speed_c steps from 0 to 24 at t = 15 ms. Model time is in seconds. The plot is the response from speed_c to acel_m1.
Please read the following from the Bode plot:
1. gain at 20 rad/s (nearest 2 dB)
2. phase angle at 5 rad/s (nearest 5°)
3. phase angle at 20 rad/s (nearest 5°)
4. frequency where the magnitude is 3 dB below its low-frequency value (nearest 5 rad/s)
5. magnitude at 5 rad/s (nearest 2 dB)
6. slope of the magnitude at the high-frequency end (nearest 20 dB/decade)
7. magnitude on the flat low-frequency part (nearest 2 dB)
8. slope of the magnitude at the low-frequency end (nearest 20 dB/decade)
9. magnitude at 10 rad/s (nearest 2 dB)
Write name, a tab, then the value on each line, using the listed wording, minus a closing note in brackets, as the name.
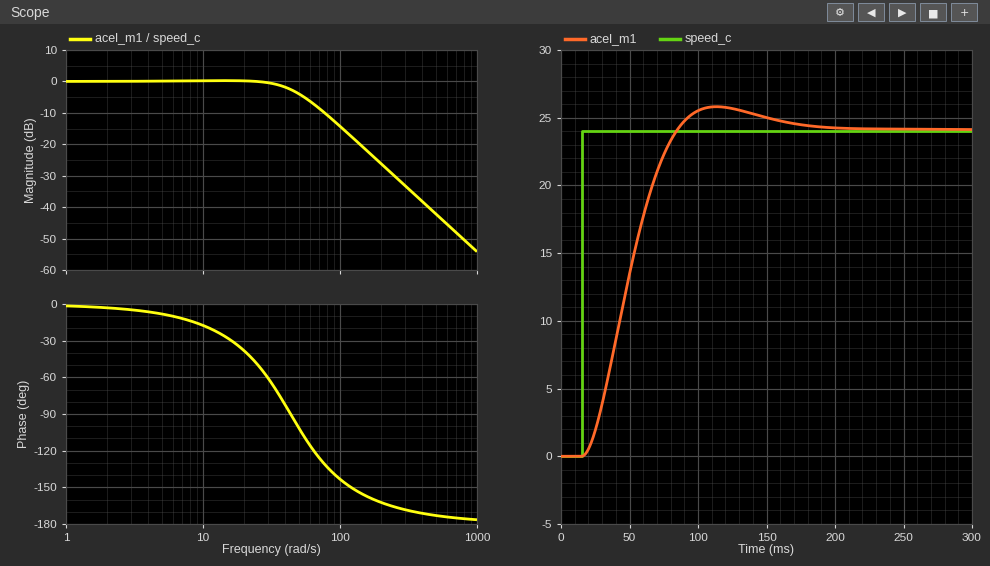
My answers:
gain at 20 rad/s	0 dB
phase angle at 5 rad/s	-10°
phase angle at 20 rad/s	-40°
frequency where the magnitude is 3 dB below its low-frequency value	45 rad/s
magnitude at 5 rad/s	0 dB
slope of the magnitude at the high-frequency end	-40 dB/decade
magnitude on the flat low-frequency part	0 dB
slope of the magnitude at the low-frequency end	0 dB/decade
magnitude at 10 rad/s	0 dB
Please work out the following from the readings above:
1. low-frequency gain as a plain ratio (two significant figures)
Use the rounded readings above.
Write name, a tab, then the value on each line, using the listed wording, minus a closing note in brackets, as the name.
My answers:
low-frequency gain as a plain ratio	1.0
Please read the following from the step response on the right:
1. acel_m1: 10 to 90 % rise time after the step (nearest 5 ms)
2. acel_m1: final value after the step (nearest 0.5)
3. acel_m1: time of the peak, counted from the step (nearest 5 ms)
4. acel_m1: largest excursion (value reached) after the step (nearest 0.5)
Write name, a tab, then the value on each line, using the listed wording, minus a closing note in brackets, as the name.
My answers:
acel_m1: 10 to 90 % rise time after the step	45 ms
acel_m1: final value after the step	24.0
acel_m1: time of the peak, counted from the step	100 ms
acel_m1: largest excursion (value reached) after the step	26.0
